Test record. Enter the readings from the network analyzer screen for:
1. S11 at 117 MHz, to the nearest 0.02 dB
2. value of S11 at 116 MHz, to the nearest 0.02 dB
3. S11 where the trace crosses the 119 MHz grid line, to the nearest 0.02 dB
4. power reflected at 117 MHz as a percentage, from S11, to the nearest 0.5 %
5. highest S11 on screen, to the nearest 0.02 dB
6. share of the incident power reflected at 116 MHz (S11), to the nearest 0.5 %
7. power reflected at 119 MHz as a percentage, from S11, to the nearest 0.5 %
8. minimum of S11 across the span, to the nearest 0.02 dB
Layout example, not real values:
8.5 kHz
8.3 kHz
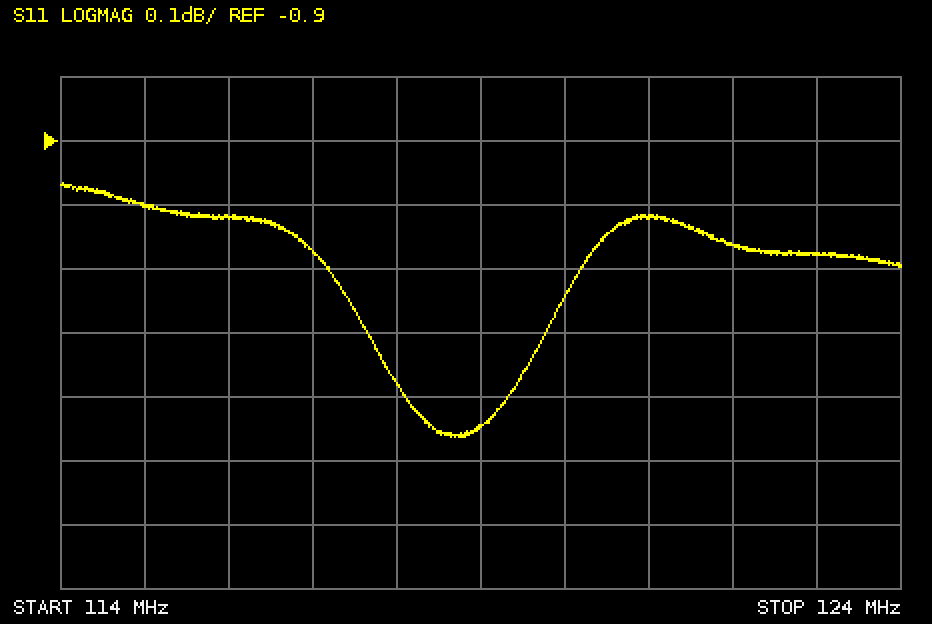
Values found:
-1.08 dB
-1.02 dB
-1.34 dB
78.0 %
-0.96 dB
79.0 %
73.5 %
-1.36 dB
